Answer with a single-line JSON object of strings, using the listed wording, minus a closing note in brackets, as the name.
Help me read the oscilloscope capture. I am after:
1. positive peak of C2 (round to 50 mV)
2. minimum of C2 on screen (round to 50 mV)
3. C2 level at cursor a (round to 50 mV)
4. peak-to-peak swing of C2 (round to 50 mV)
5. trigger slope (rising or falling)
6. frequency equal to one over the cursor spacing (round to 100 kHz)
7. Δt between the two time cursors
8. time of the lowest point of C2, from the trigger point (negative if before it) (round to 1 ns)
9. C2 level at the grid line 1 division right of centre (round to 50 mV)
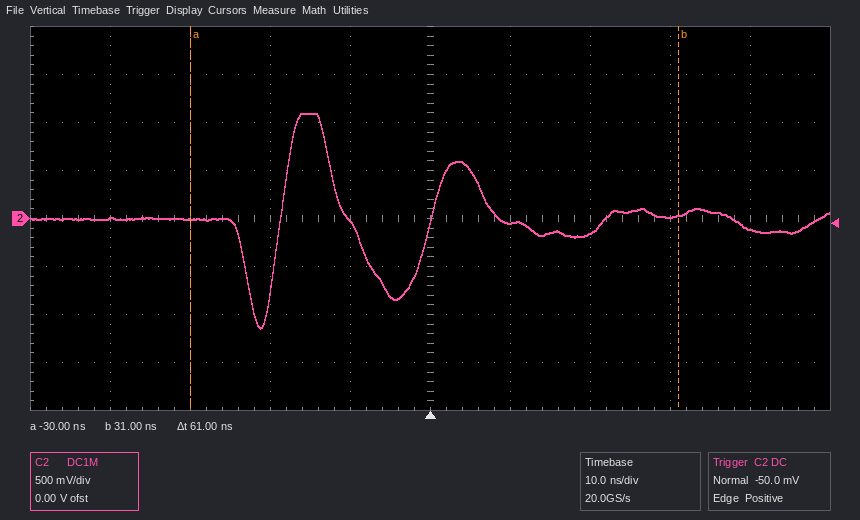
{"positive peak of C2": "1.10 V", "minimum of C2 on screen": "-1.15 V", "C2 level at cursor a": "0 mV", "peak-to-peak swing of C2": "2.25 V", "trigger slope": "rising", "frequency equal to one over the cursor spacing": "16.4 MHz", "Δt between the two time cursors": "61 ns", "time of the lowest point of C2, from the trigger point (negative if before it)": "-21 ns", "C2 level at the grid line 1 division right of centre": "-50 mV"}
